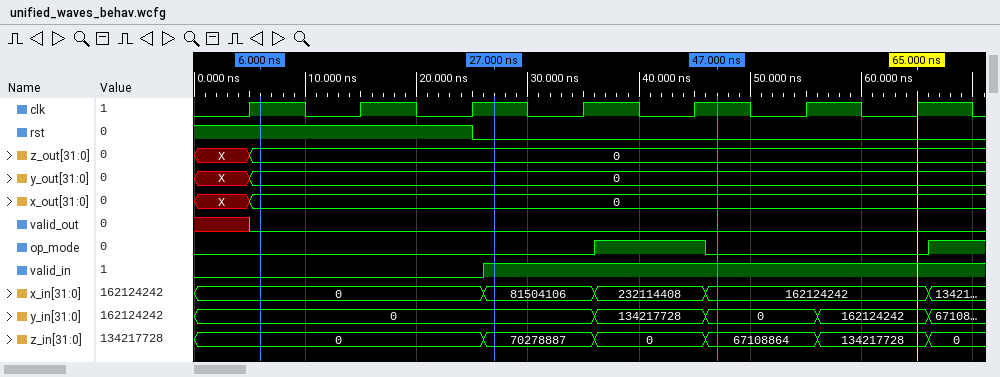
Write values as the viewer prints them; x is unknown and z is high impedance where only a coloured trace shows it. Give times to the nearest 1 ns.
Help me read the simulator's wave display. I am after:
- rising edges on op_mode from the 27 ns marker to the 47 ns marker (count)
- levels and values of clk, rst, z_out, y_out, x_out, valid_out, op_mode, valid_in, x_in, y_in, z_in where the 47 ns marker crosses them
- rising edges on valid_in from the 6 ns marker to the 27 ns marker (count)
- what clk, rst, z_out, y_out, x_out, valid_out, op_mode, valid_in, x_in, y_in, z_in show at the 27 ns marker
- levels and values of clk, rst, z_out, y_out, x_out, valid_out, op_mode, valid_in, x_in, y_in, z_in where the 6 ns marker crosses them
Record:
1
clk=1, rst=0, z_out=0, y_out=0, x_out=0, valid_out=0, op_mode=0, valid_in=1, x_in=162124242, y_in=0, z_in=67108864
1
clk=1, rst=0, z_out=0, y_out=0, x_out=0, valid_out=0, op_mode=0, valid_in=1, x_in=81504106, y_in=0, z_in=70278887
clk=1, rst=1, z_out=0, y_out=0, x_out=0, valid_out=0, op_mode=0, valid_in=0, x_in=0, y_in=0, z_in=0
